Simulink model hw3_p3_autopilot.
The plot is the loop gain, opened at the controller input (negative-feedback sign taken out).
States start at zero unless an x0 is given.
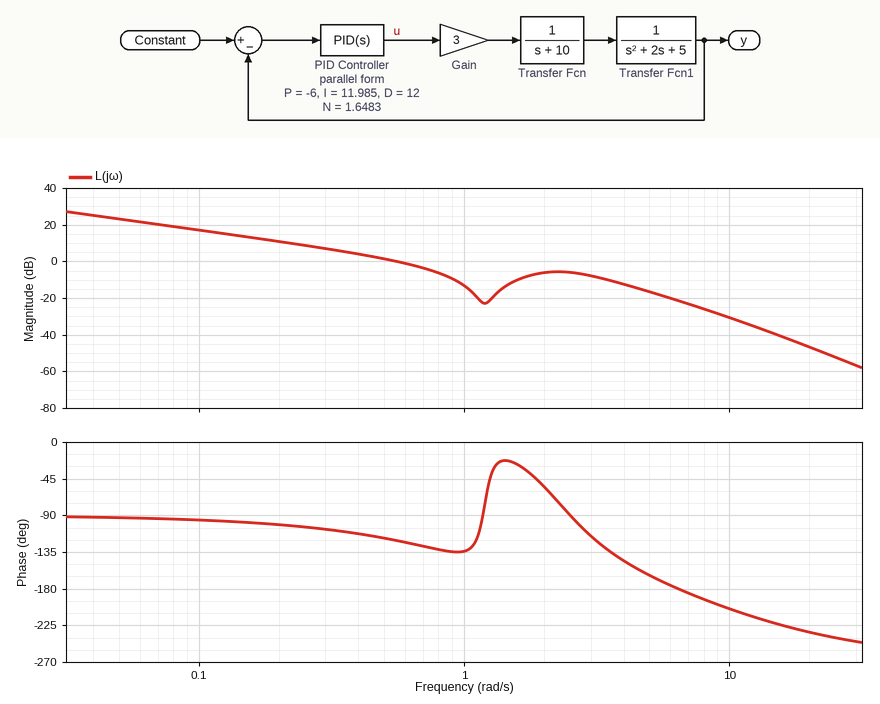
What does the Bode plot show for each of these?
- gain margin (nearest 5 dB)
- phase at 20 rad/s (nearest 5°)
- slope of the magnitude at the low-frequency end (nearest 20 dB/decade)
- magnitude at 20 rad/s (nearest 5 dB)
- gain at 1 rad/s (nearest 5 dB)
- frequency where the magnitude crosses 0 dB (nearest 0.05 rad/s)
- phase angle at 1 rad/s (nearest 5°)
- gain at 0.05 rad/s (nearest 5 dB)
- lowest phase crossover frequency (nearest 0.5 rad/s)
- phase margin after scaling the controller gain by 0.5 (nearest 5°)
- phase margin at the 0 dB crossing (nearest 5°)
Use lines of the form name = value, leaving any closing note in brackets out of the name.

gain margin = 20 dB
phase at 20 rad/s = -235°
slope of the magnitude at the low-frequency end = -20 dB/decade
magnitude at 20 rad/s = -45 dB
gain at 1 rad/s = -15 dB
frequency where the magnitude crosses 0 dB = 0.55 rad/s
phase angle at 1 rad/s = -135°
gain at 0.05 rad/s = 25 dB
lowest phase crossover frequency = 6.5 rad/s
phase margin after scaling the controller gain by 0.5 = 70°
phase margin at the 0 dB crossing = 60°
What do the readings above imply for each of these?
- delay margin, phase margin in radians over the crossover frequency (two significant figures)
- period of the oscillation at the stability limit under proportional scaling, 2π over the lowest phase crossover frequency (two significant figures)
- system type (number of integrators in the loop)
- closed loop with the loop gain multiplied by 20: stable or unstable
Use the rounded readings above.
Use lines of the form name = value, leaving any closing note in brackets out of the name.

delay margin, phase margin in radians over the crossover frequency = 1.9 s
period of the oscillation at the stability limit under proportional scaling, 2π over the lowest phase crossover frequency = 0.97 s
system type = 1
closed loop with the loop gain multiplied by 20: stable or unstable = unstable
